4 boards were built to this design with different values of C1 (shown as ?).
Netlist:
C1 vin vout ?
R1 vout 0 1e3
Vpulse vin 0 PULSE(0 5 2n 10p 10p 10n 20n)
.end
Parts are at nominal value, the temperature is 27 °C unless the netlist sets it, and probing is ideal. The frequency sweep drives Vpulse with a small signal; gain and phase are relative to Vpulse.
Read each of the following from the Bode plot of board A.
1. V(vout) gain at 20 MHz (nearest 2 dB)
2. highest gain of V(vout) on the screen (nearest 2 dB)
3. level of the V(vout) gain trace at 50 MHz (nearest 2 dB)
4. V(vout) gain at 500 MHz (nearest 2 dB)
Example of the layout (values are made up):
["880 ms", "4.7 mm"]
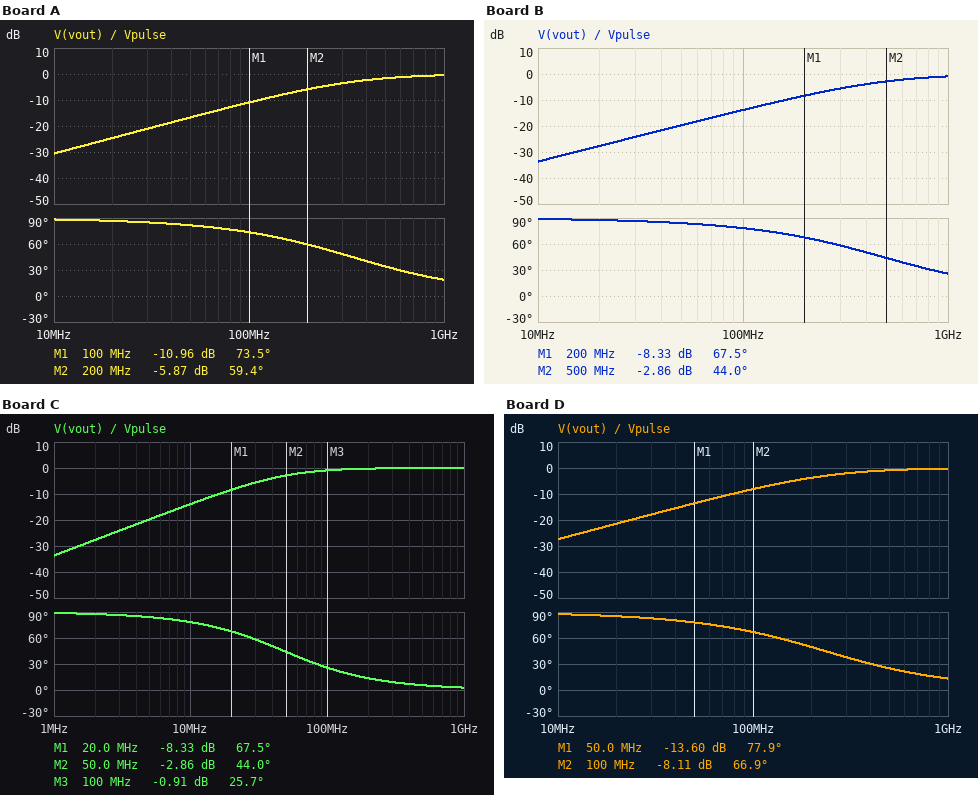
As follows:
["-24 dB", "0 dB", "-16 dB", "-2 dB"]
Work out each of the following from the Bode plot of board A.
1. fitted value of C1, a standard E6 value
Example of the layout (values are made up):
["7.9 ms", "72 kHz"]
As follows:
["470 fF"]
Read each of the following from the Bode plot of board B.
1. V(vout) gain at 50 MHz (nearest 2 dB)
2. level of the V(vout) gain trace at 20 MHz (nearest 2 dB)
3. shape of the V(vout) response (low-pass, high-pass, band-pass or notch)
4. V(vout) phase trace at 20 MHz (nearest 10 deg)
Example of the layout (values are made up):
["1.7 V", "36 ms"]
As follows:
["-20 dB", "-28 dB", "high-pass", "90 deg"]
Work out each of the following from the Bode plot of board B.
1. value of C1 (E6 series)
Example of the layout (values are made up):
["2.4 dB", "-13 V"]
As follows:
["330 fF"]
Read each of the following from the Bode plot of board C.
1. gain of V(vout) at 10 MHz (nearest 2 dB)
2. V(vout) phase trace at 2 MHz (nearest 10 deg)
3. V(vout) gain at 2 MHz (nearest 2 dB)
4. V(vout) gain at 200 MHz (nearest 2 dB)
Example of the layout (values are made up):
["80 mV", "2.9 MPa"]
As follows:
["-14 dB", "90 deg", "-28 dB", "0 dB"]
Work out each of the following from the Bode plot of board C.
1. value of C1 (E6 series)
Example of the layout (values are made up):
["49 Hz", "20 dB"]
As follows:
["3.3 pF"]
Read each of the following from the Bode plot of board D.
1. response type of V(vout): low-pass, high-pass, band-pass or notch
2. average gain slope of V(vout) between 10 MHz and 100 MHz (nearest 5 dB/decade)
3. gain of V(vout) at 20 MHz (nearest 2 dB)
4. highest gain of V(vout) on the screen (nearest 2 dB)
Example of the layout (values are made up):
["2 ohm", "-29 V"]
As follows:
["high-pass", "20 dB/decade", "-22 dB", "0 dB"]
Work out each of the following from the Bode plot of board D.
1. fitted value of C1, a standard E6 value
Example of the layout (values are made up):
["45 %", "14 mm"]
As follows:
["680 fF"]
